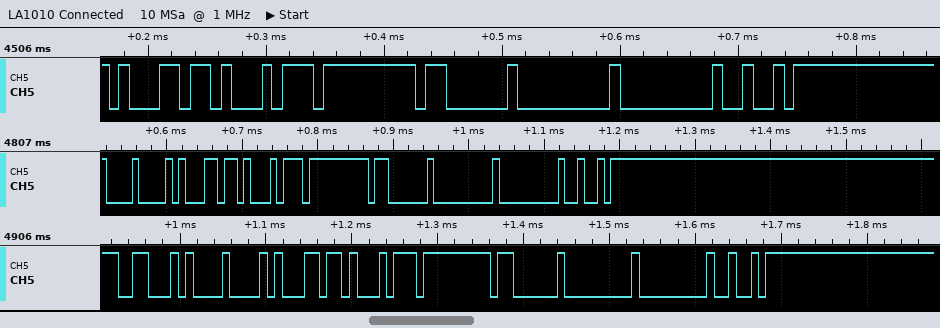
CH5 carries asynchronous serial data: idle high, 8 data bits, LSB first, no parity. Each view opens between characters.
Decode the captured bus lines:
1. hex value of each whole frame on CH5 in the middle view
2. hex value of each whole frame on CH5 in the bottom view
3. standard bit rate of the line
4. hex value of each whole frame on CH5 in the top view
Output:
08, B1, D1, FF, 03, 00, 00, D2
46, 08, B1, D1, FF, 03, 00, 00, D2
115200 baud
B1, D1, FF, 03, 00, 00, D2
